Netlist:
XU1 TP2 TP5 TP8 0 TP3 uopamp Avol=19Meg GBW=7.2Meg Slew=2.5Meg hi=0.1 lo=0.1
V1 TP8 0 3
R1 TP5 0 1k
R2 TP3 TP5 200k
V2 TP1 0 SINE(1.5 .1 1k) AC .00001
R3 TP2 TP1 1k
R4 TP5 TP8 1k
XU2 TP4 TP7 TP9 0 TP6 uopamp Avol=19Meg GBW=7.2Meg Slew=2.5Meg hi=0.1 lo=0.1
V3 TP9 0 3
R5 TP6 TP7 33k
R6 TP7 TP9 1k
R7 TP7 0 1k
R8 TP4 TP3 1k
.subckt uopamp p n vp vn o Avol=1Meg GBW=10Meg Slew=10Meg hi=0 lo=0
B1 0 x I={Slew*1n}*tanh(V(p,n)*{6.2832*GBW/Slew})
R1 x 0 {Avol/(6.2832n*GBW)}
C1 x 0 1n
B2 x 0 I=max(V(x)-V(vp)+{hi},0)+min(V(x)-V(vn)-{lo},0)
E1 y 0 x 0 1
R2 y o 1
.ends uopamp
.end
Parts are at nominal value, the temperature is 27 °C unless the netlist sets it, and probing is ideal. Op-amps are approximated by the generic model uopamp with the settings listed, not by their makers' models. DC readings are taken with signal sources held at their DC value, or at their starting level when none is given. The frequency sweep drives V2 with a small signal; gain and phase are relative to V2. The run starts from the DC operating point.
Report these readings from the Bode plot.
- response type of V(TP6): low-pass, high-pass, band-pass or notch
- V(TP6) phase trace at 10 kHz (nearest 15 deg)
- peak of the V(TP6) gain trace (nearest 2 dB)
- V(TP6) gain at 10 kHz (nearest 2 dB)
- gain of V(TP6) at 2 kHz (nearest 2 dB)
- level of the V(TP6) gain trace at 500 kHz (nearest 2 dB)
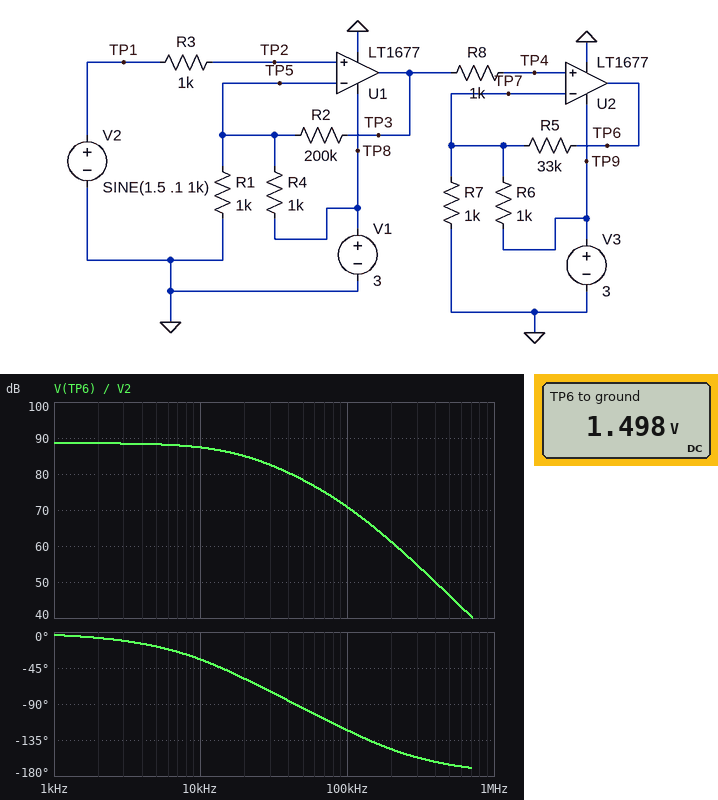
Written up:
low-pass
-30 deg
88 dB
88 dB
88 dB
46 dB
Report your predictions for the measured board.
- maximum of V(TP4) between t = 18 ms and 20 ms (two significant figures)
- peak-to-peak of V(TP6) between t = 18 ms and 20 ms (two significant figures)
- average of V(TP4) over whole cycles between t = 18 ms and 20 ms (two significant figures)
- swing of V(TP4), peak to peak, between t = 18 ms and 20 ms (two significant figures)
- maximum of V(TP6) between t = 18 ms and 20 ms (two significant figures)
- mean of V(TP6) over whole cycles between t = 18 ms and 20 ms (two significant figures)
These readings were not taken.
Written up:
2.9 V
2.8 V
1.5 V
2.8 V
2.9 V
1.5 V
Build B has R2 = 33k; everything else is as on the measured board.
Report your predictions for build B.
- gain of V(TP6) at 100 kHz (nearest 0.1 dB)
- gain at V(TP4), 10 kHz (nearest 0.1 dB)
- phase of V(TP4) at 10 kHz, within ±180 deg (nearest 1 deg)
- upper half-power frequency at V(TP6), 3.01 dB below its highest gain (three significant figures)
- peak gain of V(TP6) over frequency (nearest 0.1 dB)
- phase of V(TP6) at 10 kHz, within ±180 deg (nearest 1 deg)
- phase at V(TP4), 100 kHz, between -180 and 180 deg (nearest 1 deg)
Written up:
67.6 dB
36.5 dB
-5 deg
69.2 kHz
73.0 dB
-11 deg
-43 deg
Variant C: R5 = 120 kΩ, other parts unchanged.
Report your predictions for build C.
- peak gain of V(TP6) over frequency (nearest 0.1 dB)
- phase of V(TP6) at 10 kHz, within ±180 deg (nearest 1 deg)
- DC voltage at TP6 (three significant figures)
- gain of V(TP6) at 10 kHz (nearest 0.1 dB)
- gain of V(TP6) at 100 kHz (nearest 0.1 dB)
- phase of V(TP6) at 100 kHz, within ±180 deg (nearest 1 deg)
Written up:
99.7 dB
-48 deg
1.49 V
98.1 dB
73.8 dB
-153 deg
